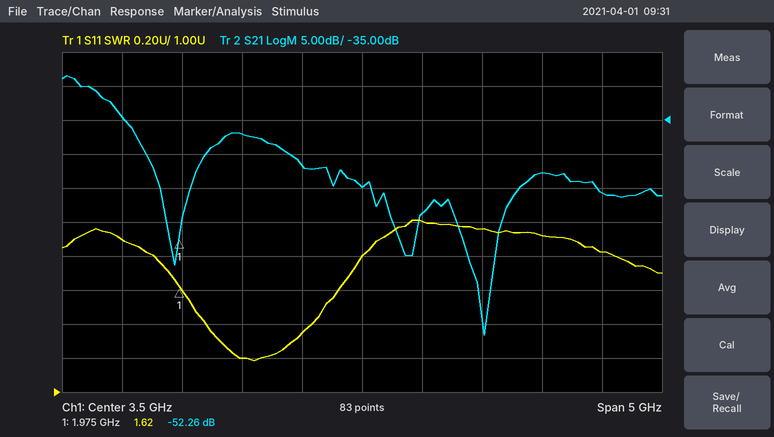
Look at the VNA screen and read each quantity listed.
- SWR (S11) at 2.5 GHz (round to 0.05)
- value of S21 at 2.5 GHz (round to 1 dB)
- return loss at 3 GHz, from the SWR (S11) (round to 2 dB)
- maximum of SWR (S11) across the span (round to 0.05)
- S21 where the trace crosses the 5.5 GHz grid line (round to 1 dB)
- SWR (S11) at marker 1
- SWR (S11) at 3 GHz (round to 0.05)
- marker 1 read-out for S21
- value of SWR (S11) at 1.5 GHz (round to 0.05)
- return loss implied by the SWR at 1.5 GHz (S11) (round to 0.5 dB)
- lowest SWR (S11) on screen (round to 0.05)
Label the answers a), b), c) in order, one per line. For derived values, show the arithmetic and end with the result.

a) 1.20
b) -37 dB
c) −20 log10((1.35 − 1)/(1.35 + 1)) ≈ 16 dB
d) 2.00
e) -46 dB
f) 1.62
g) 1.35
h) -52.26 dB
i) 1.90
j) −20 log10((1.9 − 1)/(1.9 + 1)) ≈ 10.2 dB, so 10.0 dB to the nearest 0.5 dB
k) 1.20
